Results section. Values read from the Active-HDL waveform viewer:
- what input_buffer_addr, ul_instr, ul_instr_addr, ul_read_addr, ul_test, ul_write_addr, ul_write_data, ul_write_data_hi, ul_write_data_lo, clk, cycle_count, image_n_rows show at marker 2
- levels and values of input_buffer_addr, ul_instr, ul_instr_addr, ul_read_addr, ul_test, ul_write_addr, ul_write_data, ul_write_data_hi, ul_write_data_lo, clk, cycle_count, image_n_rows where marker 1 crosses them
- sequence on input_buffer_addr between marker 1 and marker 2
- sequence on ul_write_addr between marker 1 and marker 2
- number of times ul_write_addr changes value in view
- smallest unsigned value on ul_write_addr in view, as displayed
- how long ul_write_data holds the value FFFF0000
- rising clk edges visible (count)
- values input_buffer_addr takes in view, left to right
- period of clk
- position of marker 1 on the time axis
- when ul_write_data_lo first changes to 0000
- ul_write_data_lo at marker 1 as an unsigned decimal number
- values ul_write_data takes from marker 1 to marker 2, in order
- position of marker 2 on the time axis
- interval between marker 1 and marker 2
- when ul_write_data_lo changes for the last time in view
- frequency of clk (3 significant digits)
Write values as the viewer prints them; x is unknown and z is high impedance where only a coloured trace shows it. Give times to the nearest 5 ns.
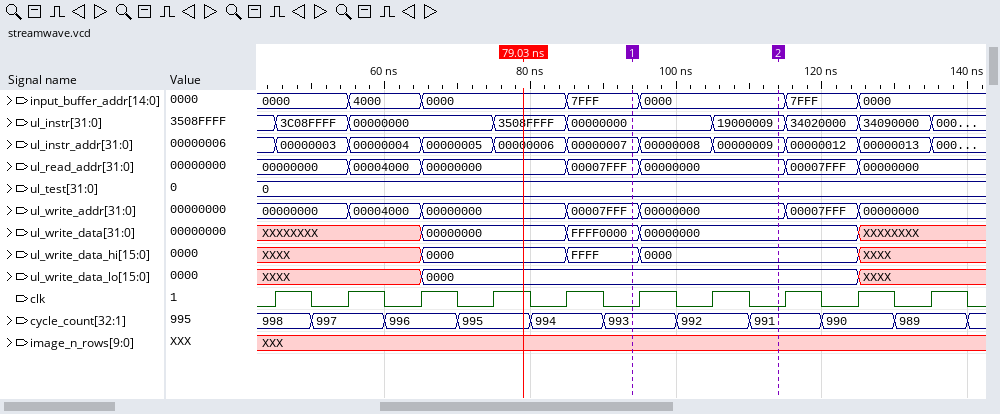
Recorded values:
input_buffer_addr=0000, ul_instr=19000009, ul_instr_addr=00000009, ul_read_addr=00000000, ul_test=0, ul_write_addr=00000000, ul_write_data=00000000, ul_write_data_hi=0000, ul_write_data_lo=0000, clk=0, cycle_count=991, image_n_rows=XXX
input_buffer_addr=7FFF, ul_instr=00000000, ul_instr_addr=00000007, ul_read_addr=00007FFF, ul_test=0, ul_write_addr=00007FFF, ul_write_data=FFFF0000, ul_write_data_hi=FFFF, ul_write_data_lo=0000, clk=0, cycle_count=993, image_n_rows=XXX
7FFF, 0000
00007FFF, 00000000
6
00000000
10 ns
10
0000, 4000, 0000, 7FFF, 0000, 7FFF, 0000
10 ns
95 ns
65 ns
0
FFFF0000, 00000000
115 ns
20 ns
125 ns
100 MHz
